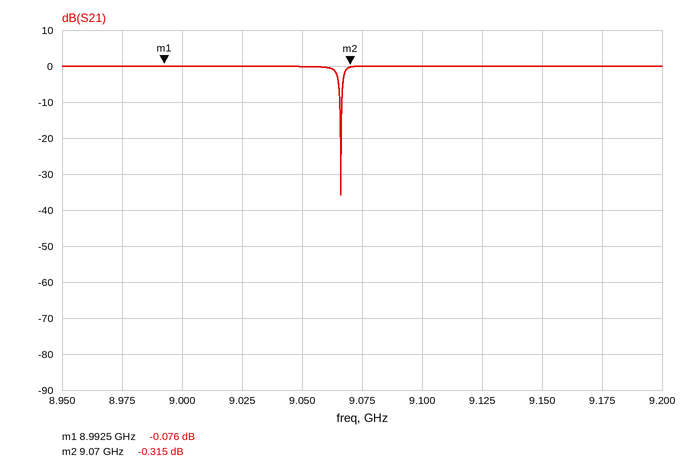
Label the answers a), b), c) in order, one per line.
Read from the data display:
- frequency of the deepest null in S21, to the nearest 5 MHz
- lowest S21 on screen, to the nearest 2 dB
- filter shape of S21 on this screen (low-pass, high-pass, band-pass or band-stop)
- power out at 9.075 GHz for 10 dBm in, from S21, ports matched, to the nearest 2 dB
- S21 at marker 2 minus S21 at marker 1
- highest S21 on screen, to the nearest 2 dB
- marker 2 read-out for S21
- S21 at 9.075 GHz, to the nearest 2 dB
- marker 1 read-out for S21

a) 9.065 GHz
b) -36 dB
c) band-stop
d) 10 dBm
e) -0.239 dB
f) 0 dB
g) -0.315 dB
h) 0 dB
i) -0.076 dB
